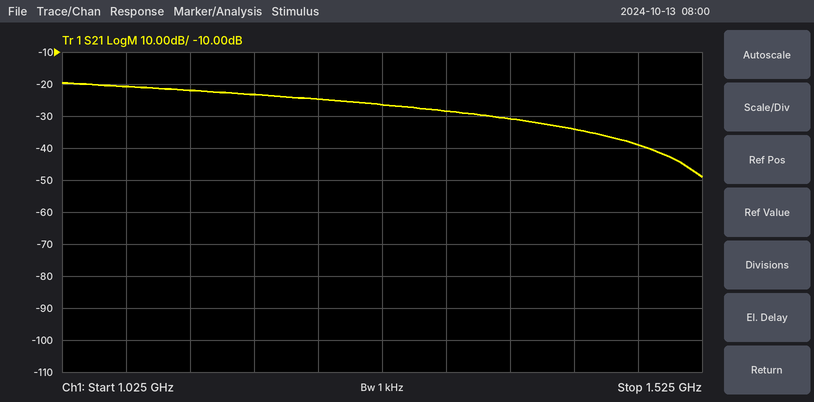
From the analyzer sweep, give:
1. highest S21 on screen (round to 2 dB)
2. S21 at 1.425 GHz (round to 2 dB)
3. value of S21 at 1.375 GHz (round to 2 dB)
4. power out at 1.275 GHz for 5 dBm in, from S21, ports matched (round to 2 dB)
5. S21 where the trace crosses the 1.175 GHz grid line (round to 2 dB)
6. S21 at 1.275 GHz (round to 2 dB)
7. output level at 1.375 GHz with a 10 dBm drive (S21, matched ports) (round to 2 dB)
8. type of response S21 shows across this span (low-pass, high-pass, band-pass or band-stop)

-20 dB
-34 dB
-30 dB
-22 dBm
-24 dB
-26 dB
-20 dBm
low-pass
